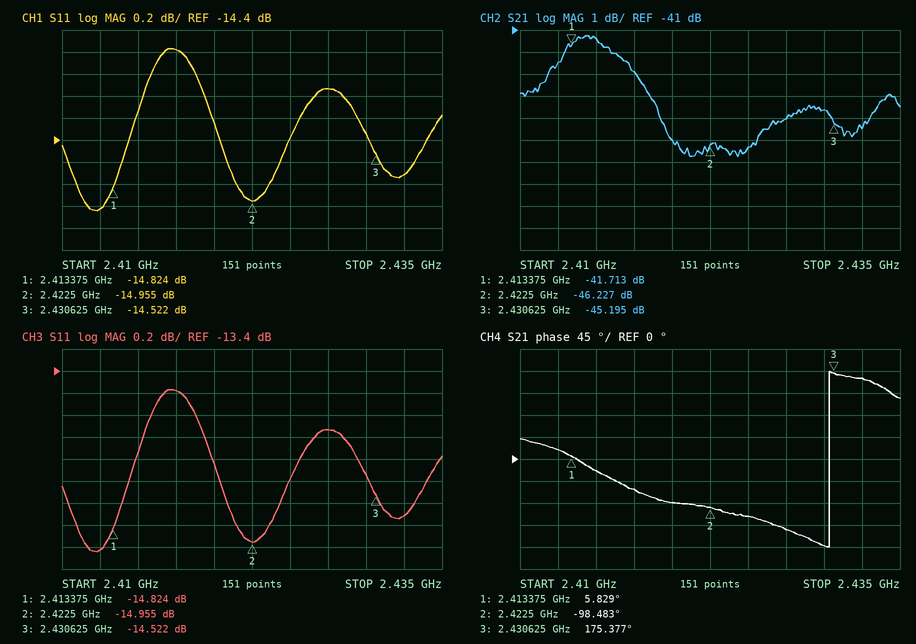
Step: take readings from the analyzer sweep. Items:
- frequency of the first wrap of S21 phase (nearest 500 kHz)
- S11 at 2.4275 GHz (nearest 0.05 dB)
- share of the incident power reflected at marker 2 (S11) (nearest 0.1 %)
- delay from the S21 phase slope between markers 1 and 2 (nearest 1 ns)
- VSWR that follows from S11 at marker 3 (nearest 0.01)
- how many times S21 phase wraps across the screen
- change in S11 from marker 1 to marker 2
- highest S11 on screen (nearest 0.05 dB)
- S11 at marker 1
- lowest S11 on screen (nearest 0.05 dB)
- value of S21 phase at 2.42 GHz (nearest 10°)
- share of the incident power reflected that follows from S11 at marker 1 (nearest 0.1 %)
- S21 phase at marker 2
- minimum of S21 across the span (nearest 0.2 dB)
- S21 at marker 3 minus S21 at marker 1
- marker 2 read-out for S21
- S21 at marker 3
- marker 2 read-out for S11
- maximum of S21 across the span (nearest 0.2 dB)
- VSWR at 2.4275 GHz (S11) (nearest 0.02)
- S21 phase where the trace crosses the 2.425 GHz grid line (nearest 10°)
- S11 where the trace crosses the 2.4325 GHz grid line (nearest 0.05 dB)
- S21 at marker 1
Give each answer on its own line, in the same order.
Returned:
2.4305 GHz
-13.95 dB
3.2 %
32 ns
1.46
1
-0.131 dB
-13.55 dB
-14.824 dB
-15.05 dB
-90°
3.3 %
-98.483°
-46.8 dB
-3.482 dB
-46.227 dB
-45.195 dB
-14.955 dB
-41.2 dB
1.50
-120°
-14.70 dB
-41.713 dB
